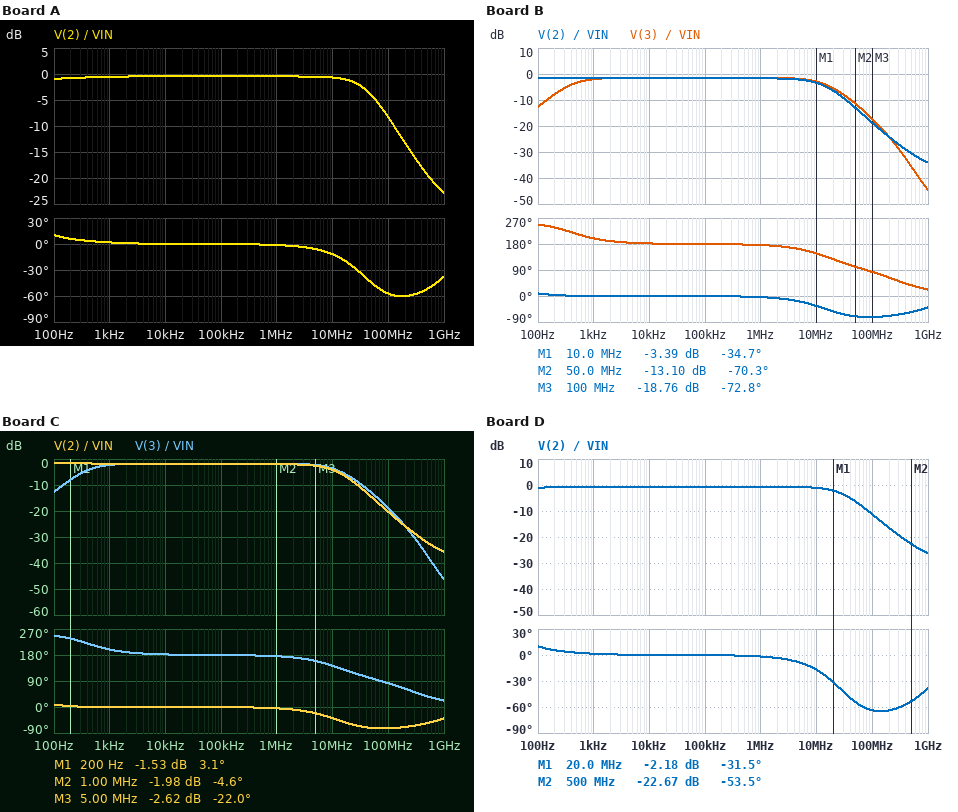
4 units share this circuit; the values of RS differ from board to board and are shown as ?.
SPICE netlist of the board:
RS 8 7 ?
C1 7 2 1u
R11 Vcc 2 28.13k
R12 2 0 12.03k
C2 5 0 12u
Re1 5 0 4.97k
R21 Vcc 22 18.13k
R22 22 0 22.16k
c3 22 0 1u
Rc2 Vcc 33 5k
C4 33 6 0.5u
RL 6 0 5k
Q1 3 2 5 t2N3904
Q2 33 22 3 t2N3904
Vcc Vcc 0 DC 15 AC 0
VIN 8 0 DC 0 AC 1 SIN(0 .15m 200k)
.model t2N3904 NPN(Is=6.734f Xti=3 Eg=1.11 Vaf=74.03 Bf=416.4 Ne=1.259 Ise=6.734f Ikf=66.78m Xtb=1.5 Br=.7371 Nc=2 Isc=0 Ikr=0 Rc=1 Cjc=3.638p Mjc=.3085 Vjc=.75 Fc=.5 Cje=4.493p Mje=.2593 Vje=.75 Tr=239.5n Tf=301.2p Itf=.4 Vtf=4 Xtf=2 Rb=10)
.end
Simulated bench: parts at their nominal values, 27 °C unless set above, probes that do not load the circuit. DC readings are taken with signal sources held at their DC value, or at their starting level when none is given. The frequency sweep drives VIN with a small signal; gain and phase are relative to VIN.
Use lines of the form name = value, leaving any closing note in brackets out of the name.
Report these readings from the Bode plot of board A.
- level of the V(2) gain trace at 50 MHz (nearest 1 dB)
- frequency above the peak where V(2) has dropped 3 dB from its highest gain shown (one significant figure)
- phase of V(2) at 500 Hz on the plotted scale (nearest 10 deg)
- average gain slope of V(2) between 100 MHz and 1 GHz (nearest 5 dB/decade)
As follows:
level of the V(2) gain trace at 50 MHz = -4 dB
frequency above the peak where V(2) has dropped 3 dB from its highest gain shown = 40 MHz
phase of V(2) at 500 Hz on the plotted scale = 0 deg
average gain slope of V(2) between 100 MHz and 1 GHz = -15 dB/decade
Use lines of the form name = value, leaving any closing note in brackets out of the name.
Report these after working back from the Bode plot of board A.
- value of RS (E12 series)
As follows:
value of RS = 180 Ω
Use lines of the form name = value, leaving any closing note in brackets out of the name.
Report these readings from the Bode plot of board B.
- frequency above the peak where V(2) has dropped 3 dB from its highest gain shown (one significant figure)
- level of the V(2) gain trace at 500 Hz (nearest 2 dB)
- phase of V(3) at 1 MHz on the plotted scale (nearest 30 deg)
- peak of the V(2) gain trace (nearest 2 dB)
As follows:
frequency above the peak where V(2) has dropped 3 dB from its highest gain shown = 10 MHz
level of the V(2) gain trace at 500 Hz = -2 dB
phase of V(3) at 1 MHz on the plotted scale = 180 deg
peak of the V(2) gain trace = -2 dB
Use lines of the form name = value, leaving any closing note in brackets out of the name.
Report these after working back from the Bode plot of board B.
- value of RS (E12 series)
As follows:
value of RS = 680 Ω
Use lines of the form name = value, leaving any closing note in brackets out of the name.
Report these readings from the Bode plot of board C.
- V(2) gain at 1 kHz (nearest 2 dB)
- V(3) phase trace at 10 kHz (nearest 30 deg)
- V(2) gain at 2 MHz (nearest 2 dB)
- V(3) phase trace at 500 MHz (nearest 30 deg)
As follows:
V(2) gain at 1 kHz = -2 dB
V(3) phase trace at 10 kHz = 180 deg
V(2) gain at 2 MHz = -2 dB
V(3) phase trace at 500 MHz = 30 deg
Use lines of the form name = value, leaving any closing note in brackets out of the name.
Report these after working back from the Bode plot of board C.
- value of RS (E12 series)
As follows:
value of RS = 820 Ω
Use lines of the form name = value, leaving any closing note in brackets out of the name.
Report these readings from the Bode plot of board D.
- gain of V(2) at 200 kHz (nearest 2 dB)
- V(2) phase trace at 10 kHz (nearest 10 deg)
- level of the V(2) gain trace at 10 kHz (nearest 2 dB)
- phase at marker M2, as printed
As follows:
gain of V(2) at 200 kHz = 0 dB
V(2) phase trace at 10 kHz = 0 deg
level of the V(2) gain trace at 10 kHz = 0 dB
phase at marker M2, as printed = -53.5 deg
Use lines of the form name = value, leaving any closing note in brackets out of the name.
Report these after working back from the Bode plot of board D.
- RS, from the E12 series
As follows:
RS, from the E12 series = 270 Ω
